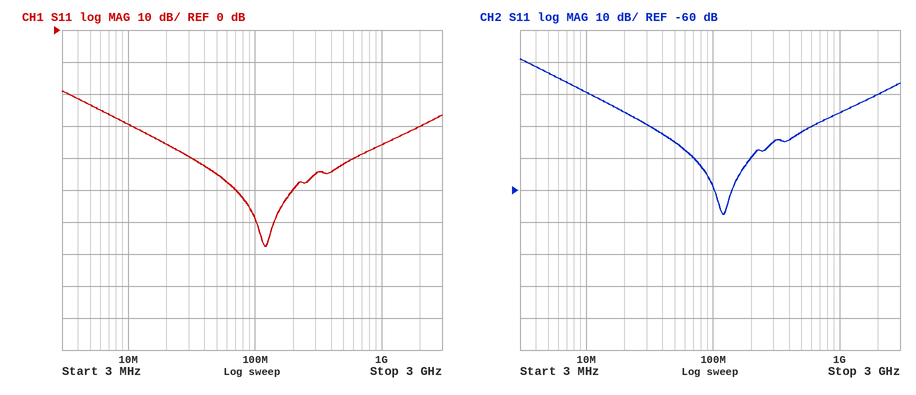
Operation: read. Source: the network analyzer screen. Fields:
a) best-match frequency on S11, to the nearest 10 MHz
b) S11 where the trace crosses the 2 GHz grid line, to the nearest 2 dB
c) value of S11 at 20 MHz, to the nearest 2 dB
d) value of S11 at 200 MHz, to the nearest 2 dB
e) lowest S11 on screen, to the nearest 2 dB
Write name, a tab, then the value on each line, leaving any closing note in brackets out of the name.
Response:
best-match frequency on S11, to the nearest 10 MHz	120 MHz
S11 where the trace crosses the 2 GHz grid line, to the nearest 2 dB	-30 dB
value of S11 at 20 MHz, to the nearest 2 dB	-36 dB
value of S11 at 200 MHz, to the nearest 2 dB	-50 dB
lowest S11 on screen, to the nearest 2 dB	-68 dB
